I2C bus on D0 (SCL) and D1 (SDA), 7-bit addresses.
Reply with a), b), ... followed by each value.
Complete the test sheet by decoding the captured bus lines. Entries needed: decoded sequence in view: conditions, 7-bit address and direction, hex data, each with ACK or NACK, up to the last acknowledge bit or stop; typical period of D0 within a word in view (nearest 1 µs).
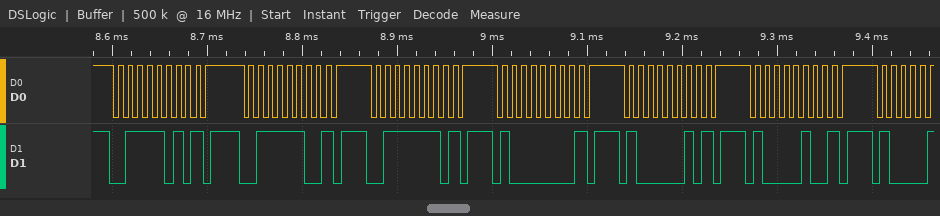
a) start, address 3D write NACK, stop, start, address 3E write NACK, stop, start, address 3F write NACK, stop, start, address 40 write NACK, stop, start, address 41 write NACK, stop, start, address 42 write NACK, stop
b) 10 µs
